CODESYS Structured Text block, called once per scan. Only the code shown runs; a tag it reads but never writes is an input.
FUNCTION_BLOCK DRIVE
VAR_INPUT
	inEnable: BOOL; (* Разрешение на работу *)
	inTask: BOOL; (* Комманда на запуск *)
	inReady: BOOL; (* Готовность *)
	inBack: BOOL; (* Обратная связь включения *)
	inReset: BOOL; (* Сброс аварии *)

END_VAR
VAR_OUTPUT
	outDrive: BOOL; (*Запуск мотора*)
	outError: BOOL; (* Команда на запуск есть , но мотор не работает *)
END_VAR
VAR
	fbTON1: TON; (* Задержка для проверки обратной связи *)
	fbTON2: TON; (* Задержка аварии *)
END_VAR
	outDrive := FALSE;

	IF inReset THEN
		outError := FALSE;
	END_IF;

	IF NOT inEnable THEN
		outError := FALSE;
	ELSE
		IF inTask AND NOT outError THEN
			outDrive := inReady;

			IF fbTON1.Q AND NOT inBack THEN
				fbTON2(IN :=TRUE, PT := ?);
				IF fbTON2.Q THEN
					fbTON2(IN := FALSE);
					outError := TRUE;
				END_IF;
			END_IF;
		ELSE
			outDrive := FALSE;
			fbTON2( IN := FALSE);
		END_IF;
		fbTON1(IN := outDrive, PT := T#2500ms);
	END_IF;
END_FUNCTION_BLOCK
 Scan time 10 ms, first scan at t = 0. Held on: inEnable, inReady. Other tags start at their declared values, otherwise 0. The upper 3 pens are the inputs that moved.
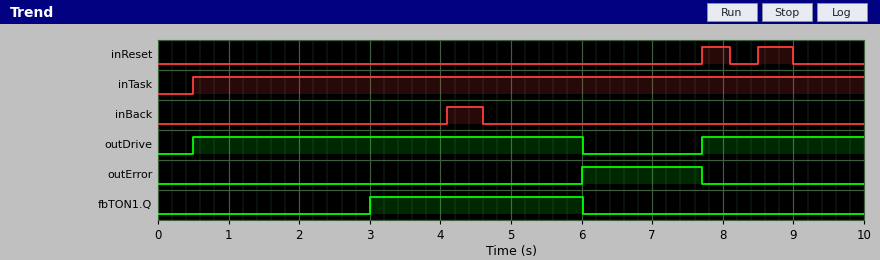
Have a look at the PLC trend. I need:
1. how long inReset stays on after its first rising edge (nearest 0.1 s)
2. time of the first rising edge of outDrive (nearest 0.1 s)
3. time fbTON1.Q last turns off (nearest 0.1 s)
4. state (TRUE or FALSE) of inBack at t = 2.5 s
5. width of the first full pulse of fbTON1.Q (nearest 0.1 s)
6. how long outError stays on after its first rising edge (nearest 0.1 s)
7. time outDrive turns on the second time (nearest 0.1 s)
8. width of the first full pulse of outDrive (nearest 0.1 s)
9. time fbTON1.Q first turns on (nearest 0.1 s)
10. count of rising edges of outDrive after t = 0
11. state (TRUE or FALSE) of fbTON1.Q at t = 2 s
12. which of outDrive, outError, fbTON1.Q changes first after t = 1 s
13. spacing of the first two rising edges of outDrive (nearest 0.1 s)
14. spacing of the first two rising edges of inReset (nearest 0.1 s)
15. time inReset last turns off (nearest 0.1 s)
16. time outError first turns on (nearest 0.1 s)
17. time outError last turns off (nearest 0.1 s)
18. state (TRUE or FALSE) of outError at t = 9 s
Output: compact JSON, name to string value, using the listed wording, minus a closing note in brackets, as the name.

{"how long inReset stays on after its first rising edge": "0.4 s", "time of the first rising edge of outDrive": "0.5 s", "time fbTON1.Q last turns off": "6.0 s", "state (TRUE or FALSE) of inBack at t = 2.5 s": "FALSE", "width of the first full pulse of fbTON1.Q": "3.0 s", "how long outError stays on after its first rising edge": "1.7 s", "time outDrive turns on the second time": "7.7 s", "width of the first full pulse of outDrive": "5.5 s", "time fbTON1.Q first turns on": "3.0 s", "count of rising edges of outDrive after t = 0": "2", "state (TRUE or FALSE) of fbTON1.Q at t = 2 s": "FALSE", "which of outDrive, outError, fbTON1.Q changes first after t = 1 s": "fbTON1.Q", "spacing of the first two rising edges of outDrive": "7.2 s", "spacing of the first two rising edges of inReset": "0.8 s", "time inReset last turns off": "9.0 s", "time outError first turns on": "6.0 s", "time outError last turns off": "7.7 s", "state (TRUE or FALSE) of outError at t = 9 s": "FALSE"}
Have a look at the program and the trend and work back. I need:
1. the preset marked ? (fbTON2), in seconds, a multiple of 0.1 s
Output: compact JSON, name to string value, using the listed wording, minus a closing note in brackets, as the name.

{"the preset marked ? (fbTON2), in seconds, a multiple of 0.1 s": "3.0 s"}
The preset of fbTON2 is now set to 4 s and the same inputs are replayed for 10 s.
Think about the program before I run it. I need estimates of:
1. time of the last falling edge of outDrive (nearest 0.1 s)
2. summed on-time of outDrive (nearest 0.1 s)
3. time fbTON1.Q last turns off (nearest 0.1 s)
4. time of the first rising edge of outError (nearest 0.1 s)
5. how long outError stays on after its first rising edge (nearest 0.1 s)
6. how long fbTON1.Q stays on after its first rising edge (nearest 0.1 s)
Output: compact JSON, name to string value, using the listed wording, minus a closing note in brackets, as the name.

{"time of the last falling edge of outDrive": "7.0 s", "summed on-time of outDrive": "8.8 s", "time fbTON1.Q last turns off": "7.0 s", "time of the first rising edge of outError": "7.0 s", "how long outError stays on after its first rising edge": "0.7 s", "how long fbTON1.Q stays on after its first rising edge": "4.0 s"}
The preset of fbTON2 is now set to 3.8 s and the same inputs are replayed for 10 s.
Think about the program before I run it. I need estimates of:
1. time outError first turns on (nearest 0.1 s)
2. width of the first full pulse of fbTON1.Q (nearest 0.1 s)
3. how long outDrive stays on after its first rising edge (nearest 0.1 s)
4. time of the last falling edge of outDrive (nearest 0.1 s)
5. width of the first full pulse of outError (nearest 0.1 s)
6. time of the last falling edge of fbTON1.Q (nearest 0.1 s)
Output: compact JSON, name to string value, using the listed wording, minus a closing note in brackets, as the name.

{"time outError first turns on": "6.8 s", "width of the first full pulse of fbTON1.Q": "3.8 s", "how long outDrive stays on after its first rising edge": "6.3 s", "time of the last falling edge of outDrive": "6.8 s", "width of the first full pulse of outError": "0.9 s", "time of the last falling edge of fbTON1.Q": "6.8 s"}
